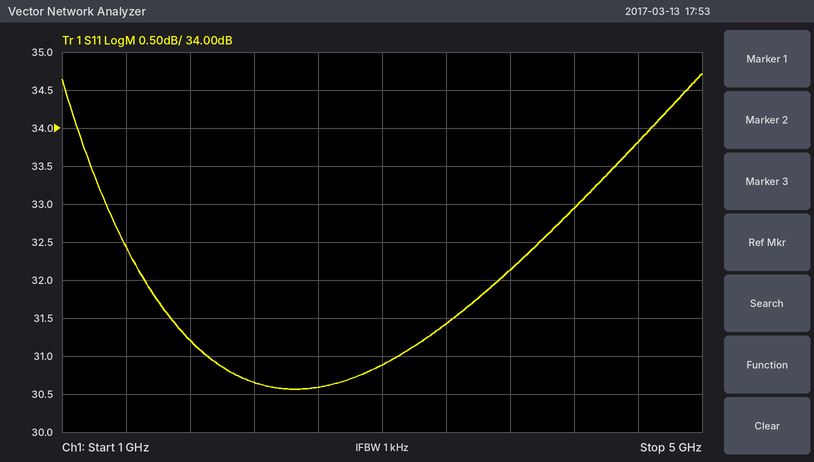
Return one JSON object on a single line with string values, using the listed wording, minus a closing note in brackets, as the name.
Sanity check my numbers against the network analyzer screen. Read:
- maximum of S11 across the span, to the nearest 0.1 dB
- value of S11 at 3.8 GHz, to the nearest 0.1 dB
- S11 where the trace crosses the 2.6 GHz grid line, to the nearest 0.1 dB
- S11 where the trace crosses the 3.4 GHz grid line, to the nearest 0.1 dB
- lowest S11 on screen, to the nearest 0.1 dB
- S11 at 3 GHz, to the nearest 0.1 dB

{"maximum of S11 across the span, to the nearest 0.1 dB": "34.7 dB", "value of S11 at 3.8 GHz, to the nearest 0.1 dB": "32.1 dB", "S11 where the trace crosses the 2.6 GHz grid line, to the nearest 0.1 dB": "30.6 dB", "S11 where the trace crosses the 3.4 GHz grid line, to the nearest 0.1 dB": "31.4 dB", "lowest S11 on screen, to the nearest 0.1 dB": "30.6 dB", "S11 at 3 GHz, to the nearest 0.1 dB": "30.9 dB"}
